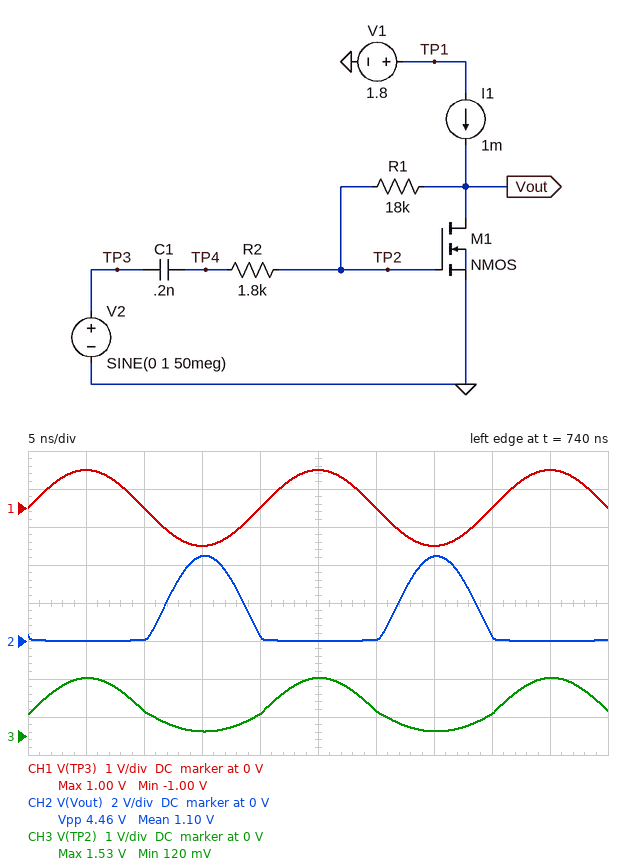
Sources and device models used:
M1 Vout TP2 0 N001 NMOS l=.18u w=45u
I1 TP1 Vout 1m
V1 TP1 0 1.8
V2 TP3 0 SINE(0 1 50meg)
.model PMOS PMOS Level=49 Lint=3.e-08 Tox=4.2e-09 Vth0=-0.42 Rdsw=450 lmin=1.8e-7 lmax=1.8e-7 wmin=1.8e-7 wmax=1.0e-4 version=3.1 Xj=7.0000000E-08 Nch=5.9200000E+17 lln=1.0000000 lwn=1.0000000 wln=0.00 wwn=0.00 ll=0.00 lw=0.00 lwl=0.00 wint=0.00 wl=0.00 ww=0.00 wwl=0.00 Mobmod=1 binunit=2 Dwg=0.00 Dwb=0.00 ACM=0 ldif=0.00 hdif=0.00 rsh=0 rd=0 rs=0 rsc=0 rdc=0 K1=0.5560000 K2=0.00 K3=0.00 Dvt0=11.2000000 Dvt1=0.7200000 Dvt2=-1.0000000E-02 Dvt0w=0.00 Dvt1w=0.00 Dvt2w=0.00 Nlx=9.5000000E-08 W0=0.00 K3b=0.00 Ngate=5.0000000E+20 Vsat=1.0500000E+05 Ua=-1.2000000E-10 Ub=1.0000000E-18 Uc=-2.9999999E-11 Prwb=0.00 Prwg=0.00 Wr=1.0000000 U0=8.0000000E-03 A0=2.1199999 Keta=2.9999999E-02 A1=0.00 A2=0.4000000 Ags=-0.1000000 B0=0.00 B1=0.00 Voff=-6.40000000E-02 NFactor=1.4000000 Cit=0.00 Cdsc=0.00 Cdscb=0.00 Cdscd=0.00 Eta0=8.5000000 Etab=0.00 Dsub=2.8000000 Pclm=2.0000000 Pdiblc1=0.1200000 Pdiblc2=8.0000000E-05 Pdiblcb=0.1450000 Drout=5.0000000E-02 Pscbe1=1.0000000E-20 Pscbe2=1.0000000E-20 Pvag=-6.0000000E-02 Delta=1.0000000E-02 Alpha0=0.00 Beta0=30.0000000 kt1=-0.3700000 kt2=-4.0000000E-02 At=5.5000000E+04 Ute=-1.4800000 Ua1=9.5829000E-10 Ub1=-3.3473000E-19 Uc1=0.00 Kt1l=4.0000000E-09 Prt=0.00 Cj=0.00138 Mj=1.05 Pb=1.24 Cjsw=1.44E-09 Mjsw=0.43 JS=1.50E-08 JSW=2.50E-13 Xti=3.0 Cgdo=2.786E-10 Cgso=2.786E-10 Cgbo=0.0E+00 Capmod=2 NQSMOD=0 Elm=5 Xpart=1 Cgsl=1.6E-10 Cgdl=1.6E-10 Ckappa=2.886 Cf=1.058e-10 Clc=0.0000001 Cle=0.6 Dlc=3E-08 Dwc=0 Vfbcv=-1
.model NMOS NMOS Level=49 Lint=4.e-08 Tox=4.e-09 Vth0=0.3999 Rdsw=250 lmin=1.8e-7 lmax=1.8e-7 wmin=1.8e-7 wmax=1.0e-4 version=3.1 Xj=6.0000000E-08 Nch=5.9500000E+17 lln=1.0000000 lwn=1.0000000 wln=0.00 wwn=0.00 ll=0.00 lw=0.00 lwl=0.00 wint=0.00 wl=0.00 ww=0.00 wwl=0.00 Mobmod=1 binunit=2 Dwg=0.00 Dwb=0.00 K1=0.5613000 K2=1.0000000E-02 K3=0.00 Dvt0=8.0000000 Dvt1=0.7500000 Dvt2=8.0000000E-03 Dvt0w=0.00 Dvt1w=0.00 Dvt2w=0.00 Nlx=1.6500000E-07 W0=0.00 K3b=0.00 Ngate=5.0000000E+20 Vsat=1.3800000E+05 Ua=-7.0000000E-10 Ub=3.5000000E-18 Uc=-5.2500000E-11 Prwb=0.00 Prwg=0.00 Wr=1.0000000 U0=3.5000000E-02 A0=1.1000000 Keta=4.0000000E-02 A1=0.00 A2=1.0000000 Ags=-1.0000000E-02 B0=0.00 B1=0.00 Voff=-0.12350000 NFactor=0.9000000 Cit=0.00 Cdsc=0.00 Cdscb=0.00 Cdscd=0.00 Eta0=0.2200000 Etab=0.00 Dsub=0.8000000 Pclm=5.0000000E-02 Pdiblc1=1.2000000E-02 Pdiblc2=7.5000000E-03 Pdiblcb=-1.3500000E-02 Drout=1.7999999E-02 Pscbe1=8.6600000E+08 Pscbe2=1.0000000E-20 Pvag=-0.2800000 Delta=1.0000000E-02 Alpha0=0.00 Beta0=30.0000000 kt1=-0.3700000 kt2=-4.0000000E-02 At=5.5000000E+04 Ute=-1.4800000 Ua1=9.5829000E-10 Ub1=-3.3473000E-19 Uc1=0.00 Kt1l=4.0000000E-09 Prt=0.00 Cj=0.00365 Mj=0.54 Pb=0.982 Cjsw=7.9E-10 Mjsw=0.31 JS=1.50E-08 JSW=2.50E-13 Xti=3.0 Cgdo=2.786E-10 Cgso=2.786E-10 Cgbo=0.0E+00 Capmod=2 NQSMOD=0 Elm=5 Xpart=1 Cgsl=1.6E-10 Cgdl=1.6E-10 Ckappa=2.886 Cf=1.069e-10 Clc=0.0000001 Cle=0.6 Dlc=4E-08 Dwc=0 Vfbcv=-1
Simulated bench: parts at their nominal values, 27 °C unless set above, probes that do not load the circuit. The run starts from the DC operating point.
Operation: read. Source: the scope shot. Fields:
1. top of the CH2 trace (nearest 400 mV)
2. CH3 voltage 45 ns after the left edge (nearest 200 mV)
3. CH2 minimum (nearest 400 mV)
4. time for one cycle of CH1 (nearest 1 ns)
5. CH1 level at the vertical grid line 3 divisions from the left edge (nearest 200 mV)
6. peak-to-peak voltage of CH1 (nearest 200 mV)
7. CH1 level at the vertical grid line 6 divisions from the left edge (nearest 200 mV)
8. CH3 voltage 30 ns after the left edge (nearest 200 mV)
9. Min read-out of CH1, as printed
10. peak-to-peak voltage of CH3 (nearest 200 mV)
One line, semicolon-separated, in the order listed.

4.4 V; 1.6 V; 0 V; 20 ns; -1.0 V; 2.0 V; 0 V; 600 mV; -1.00 V; 1.4 V
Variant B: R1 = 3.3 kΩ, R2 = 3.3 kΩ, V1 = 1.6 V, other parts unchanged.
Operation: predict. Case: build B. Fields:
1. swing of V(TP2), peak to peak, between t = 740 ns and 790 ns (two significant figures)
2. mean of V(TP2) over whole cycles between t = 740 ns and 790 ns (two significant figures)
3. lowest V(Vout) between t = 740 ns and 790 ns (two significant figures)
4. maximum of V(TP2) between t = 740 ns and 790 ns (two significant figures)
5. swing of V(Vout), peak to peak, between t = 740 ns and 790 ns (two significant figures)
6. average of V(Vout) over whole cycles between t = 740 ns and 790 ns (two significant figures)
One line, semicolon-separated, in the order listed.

400 mV; 540 mV; 41 mV; 780 mV; 1.2 V; 550 mV
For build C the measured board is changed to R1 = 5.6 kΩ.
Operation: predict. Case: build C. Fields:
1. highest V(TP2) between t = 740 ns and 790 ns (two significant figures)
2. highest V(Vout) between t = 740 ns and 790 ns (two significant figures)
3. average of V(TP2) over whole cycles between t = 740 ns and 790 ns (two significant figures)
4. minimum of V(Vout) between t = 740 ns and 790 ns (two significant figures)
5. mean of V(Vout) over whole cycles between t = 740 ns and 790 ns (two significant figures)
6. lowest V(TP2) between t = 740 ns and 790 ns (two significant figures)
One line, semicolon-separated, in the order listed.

1.2 V; 2.3 V; 670 mV; 23 mV; 790 mV; 280 mV
